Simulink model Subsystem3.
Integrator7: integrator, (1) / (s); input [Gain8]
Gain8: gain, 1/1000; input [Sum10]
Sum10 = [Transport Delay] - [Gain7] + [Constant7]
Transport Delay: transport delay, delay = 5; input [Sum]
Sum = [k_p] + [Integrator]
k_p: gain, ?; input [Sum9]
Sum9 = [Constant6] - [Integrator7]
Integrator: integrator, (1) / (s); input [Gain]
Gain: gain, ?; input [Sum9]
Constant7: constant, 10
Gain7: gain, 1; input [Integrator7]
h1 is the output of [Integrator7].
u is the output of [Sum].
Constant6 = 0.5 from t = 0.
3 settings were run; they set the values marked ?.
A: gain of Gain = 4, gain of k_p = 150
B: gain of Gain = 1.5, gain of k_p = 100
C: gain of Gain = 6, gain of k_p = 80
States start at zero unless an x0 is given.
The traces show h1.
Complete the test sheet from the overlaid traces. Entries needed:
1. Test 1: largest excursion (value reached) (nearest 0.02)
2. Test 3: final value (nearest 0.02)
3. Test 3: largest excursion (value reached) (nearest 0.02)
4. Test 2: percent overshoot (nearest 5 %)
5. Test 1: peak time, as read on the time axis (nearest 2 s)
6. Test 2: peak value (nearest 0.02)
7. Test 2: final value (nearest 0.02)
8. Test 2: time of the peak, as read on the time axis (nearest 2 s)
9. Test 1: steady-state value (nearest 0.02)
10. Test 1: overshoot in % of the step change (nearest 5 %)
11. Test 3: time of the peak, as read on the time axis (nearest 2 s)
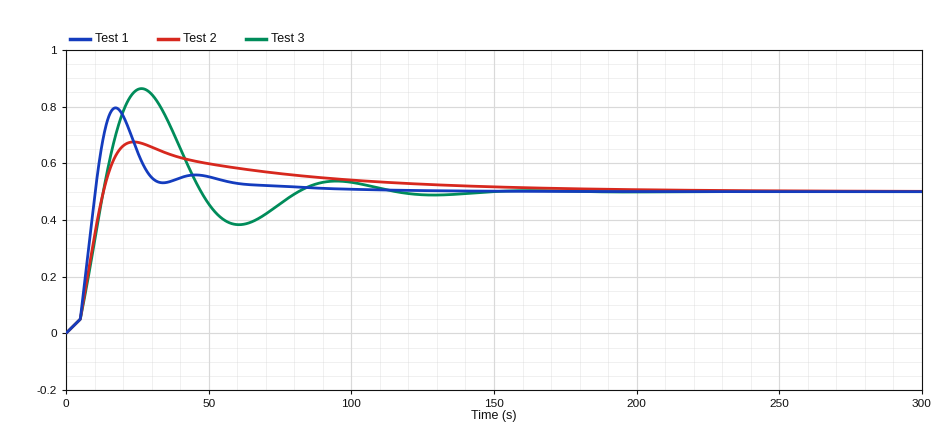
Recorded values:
0.80
0.50
0.86
35 %
18 s
0.68
0.50
24 s
0.50
60 %
26 s
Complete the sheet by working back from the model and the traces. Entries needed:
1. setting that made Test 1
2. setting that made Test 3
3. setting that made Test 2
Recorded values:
A
C
B
